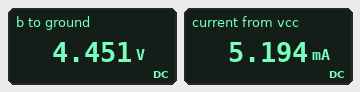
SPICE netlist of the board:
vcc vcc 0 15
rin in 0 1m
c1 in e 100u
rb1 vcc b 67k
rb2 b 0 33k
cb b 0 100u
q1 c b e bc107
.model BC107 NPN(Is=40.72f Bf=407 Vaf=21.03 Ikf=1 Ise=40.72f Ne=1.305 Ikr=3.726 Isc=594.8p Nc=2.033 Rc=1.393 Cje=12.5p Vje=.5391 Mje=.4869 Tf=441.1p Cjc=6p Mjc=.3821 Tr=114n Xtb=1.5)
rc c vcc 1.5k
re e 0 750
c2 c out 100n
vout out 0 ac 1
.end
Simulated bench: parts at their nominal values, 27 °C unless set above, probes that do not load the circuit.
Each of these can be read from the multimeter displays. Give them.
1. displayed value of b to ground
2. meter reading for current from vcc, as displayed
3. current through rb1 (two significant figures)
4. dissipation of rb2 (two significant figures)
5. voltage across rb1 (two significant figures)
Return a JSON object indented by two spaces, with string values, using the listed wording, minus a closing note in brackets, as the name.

{
  "displayed value of b to ground": "4.451 V",
  "meter reading for current from vcc, as displayed": "5.194 mA",
  "current through rb1": "160 µA",
  "dissipation of rb2": "600 µW",
  "voltage across rb1": "11 V"
}
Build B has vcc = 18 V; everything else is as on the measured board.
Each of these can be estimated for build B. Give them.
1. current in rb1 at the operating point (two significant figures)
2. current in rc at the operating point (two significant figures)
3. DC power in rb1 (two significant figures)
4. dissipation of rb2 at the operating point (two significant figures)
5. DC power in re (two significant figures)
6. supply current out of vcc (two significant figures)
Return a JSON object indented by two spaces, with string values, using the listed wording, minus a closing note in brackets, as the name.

{
  "current in rb1 at the operating point": "190 µA",
  "current in rc at the operating point": "6.2 mA",
  "DC power in rb1": "2.4 mW",
  "dissipation of rb2 at the operating point": "870 µW",
  "DC power in re": "29 mW",
  "supply current out of vcc": "6.4 mA"
}
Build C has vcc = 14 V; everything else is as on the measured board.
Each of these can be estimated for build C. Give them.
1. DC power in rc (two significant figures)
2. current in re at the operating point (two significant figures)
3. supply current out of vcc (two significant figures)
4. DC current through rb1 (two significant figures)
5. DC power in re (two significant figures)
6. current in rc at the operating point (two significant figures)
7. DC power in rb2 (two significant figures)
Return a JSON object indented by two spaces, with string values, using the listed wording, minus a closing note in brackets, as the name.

{
  "DC power in rc": "32 mW",
  "current in re at the operating point": "4.7 mA",
  "supply current out of vcc": "4.8 mA",
  "DC current through rb1": "150 µA",
  "DC power in re": "16 mW",
  "current in rc at the operating point": "4.6 mA",
  "DC power in rb2": "520 µW"
}
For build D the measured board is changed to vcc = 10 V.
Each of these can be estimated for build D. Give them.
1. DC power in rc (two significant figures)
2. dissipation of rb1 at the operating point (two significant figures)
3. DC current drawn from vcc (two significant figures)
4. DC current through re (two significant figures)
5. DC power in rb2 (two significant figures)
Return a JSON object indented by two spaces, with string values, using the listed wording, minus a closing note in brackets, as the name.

{
  "DC power in rc": "14 mW",
  "dissipation of rb1 at the operating point": "740 µW",
  "DC current drawn from vcc": "3.2 mA",
  "DC current through re": "3.1 mA",
  "DC power in rb2": "270 µW"
}
